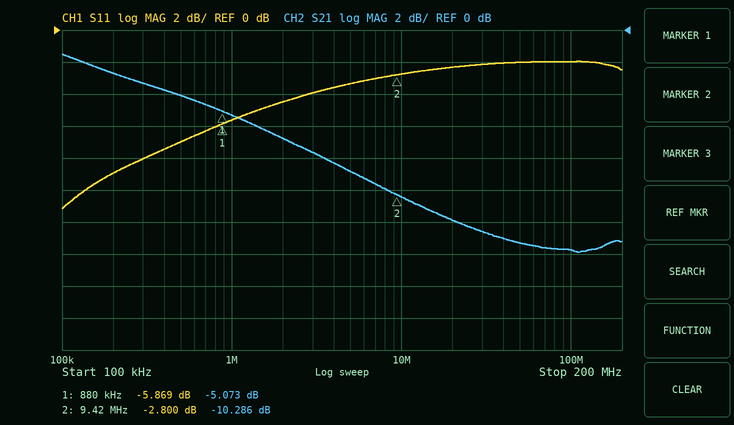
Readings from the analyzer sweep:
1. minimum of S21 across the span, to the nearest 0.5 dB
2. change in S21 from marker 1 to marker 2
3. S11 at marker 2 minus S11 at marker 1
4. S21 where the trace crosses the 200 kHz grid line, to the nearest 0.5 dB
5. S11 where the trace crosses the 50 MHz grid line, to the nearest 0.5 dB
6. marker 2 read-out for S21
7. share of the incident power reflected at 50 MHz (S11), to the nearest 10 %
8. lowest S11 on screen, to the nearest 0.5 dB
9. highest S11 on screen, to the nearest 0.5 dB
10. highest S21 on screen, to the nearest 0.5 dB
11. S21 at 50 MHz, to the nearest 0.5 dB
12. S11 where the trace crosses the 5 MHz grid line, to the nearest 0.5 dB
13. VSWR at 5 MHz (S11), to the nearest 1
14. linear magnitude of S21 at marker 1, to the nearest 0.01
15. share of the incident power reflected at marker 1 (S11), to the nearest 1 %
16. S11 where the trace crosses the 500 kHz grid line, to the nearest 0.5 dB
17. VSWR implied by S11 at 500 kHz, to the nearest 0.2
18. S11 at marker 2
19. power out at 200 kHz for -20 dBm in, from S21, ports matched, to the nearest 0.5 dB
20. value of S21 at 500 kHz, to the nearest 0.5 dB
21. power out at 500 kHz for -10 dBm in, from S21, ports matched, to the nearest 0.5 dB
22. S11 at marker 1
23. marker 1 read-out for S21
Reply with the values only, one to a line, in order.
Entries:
-14.0 dB
-5.213 dB
3.069 dB
-2.5 dB
-2.0 dB
-10.286 dB
60 %
-11.0 dB
-2.0 dB
-1.5 dB
-13.5 dB
-3.5 dB
5
0.56
26 %
-7.0 dB
2.6
-2.800 dB
-22.5 dBm
-4.0 dB
-14.0 dBm
-5.869 dB
-5.073 dB
